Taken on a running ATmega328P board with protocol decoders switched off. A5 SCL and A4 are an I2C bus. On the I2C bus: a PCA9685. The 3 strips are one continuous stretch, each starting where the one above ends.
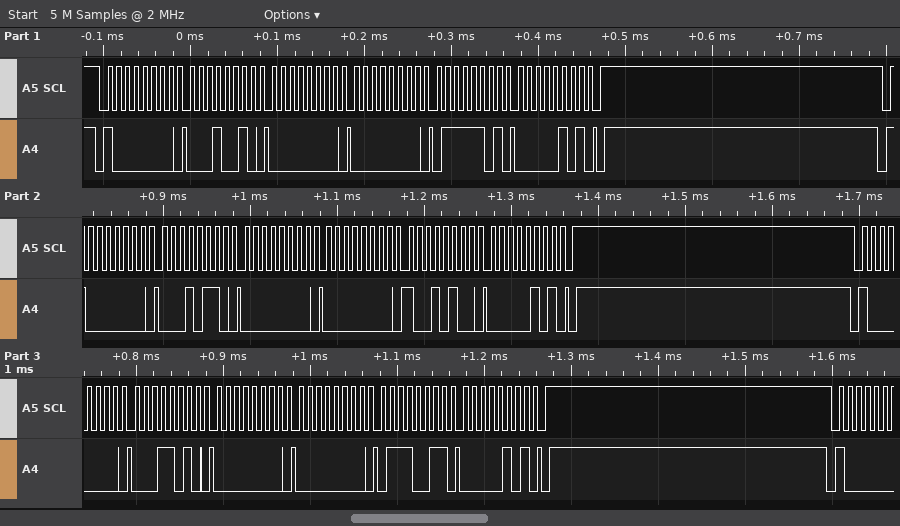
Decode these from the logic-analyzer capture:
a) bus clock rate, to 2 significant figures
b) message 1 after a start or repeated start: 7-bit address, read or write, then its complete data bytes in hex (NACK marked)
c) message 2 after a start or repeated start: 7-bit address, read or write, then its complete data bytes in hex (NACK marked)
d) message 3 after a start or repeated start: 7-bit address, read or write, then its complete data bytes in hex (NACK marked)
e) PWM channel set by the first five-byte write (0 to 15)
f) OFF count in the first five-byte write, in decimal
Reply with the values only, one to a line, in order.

100 kHz
0x40 write: 12 00 00 7D 05
0x40 write: 16 00 00 94 05
0x40 write: 1A 00 00 73 05
3
1405
